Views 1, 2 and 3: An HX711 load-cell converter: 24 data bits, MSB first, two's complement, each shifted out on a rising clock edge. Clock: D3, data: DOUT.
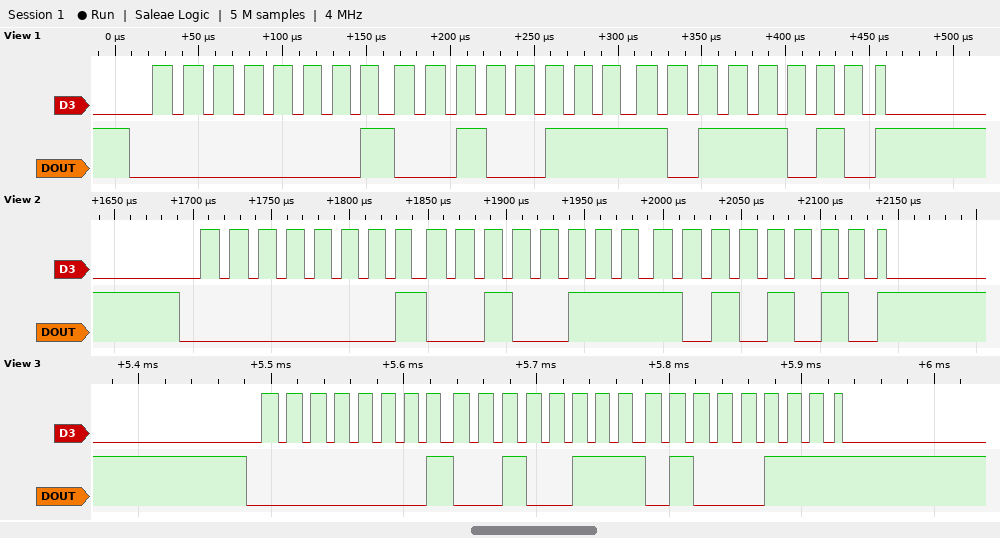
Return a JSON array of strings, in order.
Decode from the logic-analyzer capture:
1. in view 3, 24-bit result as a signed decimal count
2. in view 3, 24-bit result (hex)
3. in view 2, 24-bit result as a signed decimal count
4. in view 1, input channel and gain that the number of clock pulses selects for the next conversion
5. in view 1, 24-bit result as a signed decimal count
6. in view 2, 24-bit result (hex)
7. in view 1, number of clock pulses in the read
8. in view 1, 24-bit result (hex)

["75591", "0x012747", "75690", "channel A, gain 128", "75706", "0x0127AA", "25", "0x0127BA"]
